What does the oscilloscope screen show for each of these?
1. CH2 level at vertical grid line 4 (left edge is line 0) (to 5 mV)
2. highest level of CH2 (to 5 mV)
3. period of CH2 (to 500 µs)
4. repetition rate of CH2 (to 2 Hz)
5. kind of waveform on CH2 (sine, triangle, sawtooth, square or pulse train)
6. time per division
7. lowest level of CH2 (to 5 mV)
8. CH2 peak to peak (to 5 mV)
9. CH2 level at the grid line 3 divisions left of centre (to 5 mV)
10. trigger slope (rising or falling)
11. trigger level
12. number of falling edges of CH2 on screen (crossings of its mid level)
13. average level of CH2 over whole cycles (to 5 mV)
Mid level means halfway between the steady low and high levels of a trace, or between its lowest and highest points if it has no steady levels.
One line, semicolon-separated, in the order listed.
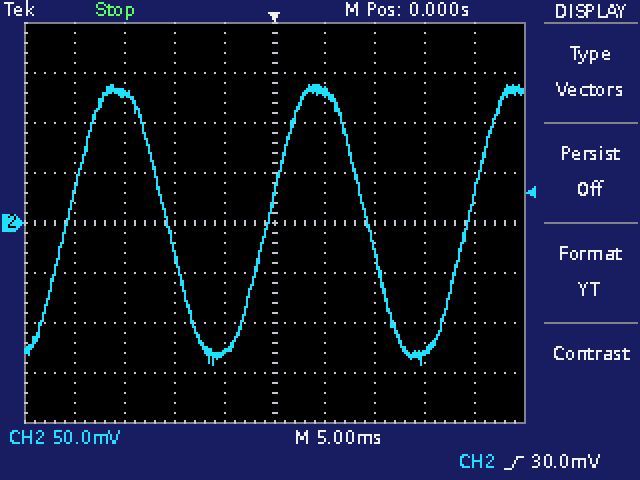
-130 mV; 140 mV; 20.0 ms; 50 Hz; sine; 5 ms; -140 mV; 280 mV; 130 mV; rising; 30.0 mV; 2; 0 mV
